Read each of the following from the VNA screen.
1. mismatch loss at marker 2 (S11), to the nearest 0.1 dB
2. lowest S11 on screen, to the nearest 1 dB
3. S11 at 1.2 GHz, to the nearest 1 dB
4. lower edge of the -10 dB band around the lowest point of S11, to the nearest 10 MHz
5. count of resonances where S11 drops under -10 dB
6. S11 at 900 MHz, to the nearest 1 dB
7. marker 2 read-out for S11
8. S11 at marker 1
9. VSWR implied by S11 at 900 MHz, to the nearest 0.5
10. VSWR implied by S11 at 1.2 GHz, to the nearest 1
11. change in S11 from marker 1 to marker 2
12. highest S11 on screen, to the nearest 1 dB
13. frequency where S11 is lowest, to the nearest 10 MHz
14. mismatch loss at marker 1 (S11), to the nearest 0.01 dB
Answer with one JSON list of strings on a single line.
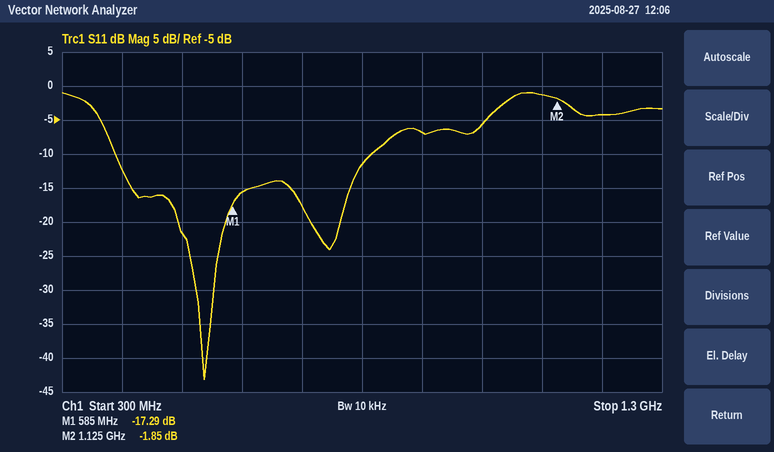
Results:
["4.6 dB", "-43 dB", "-4 dB", "390 MHz", "2", "-7 dB", "-1.85 dB", "-17.29 dB", "2.5", "4", "15.44 dB", "-1 dB", "540 MHz", "0.08 dB"]
